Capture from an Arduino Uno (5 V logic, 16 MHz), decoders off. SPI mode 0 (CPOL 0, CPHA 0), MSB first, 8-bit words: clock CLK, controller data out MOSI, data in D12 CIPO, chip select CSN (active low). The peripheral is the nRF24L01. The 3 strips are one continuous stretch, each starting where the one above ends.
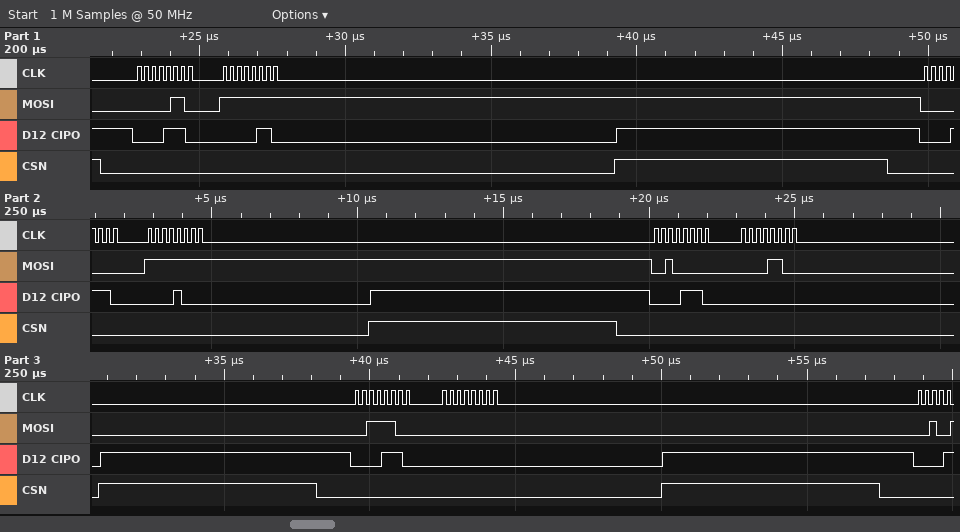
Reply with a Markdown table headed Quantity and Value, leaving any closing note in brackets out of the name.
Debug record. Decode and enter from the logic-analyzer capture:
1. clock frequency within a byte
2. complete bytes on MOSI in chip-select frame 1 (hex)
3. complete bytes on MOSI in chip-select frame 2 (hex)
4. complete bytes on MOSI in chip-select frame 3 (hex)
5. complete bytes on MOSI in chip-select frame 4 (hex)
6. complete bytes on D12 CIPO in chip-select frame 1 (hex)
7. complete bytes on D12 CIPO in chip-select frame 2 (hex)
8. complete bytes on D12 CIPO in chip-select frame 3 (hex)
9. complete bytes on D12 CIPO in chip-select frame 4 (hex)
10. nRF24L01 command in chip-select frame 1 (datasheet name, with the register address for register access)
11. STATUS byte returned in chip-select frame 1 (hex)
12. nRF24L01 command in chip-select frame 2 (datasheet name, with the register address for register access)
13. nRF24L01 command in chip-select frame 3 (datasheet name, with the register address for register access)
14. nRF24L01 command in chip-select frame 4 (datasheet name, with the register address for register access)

| Quantity | Value |
|---|---|
| clock frequency within a byte | 4 MHz |
| complete bytes on MOSI in chip-select frame 1 | 06 FF |
| complete bytes on MOSI in chip-select frame 2 | 00 FF |
| complete bytes on MOSI in chip-select frame 3 | 20 0C |
| complete bytes on MOSI in chip-select frame 4 | 3C 00 |
| complete bytes on D12 CIPO in chip-select frame 1 | 0E 06 |
| complete bytes on D12 CIPO in chip-select frame 2 | 0E 08 |
| complete bytes on D12 CIPO in chip-select frame 3 | 0E 00 |
| complete bytes on D12 CIPO in chip-select frame 4 | 0E 00 |
| nRF24L01 command in chip-select frame 1 | R_REGISTER 0x06 |
| STATUS byte returned in chip-select frame 1 | 0x0E |
| nRF24L01 command in chip-select frame 2 | R_REGISTER 0x00 |
| nRF24L01 command in chip-select frame 3 | W_REGISTER 0x00 |
| nRF24L01 command in chip-select frame 4 | W_REGISTER 0x1C |
